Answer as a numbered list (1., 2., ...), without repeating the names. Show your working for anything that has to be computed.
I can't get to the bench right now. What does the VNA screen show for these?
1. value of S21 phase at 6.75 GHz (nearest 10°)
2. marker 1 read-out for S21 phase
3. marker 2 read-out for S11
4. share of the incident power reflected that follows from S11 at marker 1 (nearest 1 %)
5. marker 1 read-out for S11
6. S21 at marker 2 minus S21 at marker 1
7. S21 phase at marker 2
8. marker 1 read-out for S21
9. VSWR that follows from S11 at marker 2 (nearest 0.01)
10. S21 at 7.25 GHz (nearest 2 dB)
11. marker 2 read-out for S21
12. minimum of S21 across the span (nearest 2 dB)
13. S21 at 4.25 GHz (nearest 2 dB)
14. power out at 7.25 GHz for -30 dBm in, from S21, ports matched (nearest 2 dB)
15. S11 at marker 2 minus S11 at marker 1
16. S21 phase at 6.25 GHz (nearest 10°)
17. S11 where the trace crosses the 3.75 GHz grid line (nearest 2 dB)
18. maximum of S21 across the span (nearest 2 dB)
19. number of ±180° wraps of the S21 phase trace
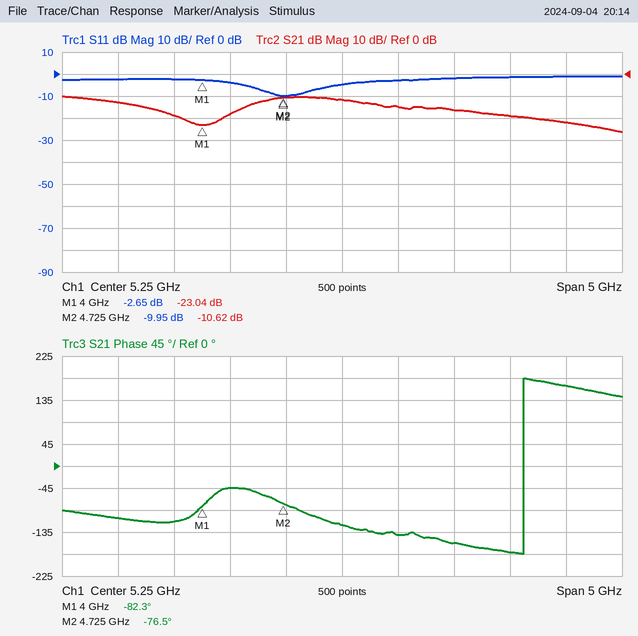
1. -180°
2. -82.3°
3. -9.95 dB
4. 10^(-2.65/10) ≈ 54 %
5. -2.65 dB
6. -10.62 − (-23.04) = 12.42 dB
7. -76.5°
8. -23.04 dB
9. (1 + 0.3181)/(1 − 0.3181) ≈ 1.93
10. -22 dB
11. -10.62 dB
12. -26 dB
13. -18 dB
14. -30 dBm + (-22 dB) = -52 dBm
15. -9.95 − (-2.65) = -7.30 dB
16. -160°
17. -2 dB
18. -10 dB
19. 1
